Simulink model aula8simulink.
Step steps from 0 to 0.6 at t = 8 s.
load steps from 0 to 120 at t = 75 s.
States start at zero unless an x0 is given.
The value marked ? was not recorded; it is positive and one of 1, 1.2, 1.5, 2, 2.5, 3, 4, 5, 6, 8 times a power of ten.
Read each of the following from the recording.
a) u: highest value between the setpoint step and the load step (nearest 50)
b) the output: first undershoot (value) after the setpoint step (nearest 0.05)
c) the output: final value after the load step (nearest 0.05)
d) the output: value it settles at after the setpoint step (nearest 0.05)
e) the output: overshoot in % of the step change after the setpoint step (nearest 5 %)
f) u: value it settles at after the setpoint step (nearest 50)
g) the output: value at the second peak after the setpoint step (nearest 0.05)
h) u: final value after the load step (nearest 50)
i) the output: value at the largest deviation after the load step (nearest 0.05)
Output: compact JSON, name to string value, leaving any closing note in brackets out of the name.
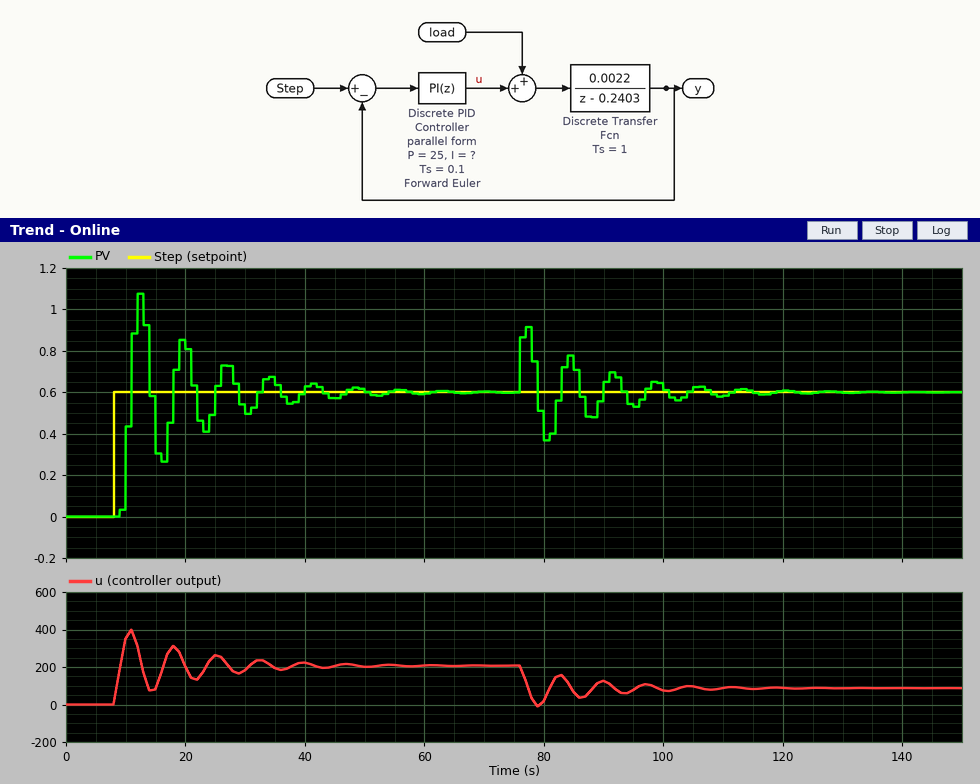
{"u: highest value between the setpoint step and the load step": "400", "the output: first undershoot (value) after the setpoint step": "0.25", "the output: final value after the load step": "0.60", "the output: value it settles at after the setpoint step": "0.60", "the output: overshoot in % of the step change after the setpoint step": "80 %", "u: value it settles at after the setpoint step": "200", "the output: value at the second peak after the setpoint step": "0.85", "u: final value after the load step": "100", "the output: value at the largest deviation after the load step": "0.90"}
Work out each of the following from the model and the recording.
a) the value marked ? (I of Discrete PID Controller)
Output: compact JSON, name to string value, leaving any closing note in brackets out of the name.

{"the value marked ?": "300"}
